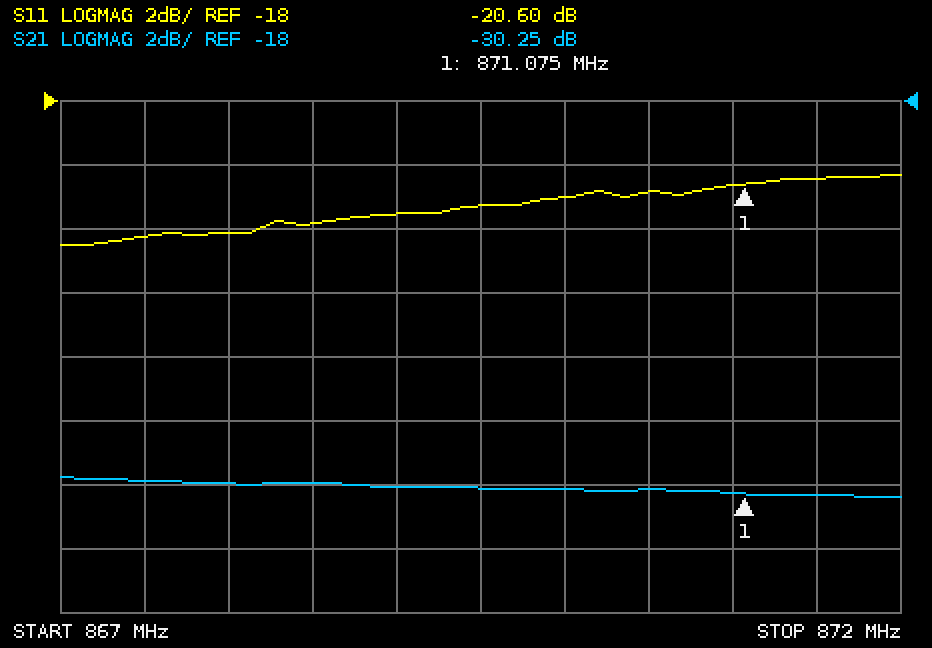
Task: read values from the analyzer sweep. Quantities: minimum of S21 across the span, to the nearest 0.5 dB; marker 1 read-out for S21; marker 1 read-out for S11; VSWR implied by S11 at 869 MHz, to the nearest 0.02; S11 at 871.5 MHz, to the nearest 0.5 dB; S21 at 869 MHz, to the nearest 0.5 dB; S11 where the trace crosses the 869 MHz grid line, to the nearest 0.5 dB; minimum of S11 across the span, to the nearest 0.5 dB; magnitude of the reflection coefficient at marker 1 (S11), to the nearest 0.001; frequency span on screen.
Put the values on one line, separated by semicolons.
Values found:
-30.5 dB; -30.25 dB; -20.60 dB; 1.18; -20.5 dB; -30.0 dB; -21.5 dB; -22.5 dB; 0.093; 5 MHz
